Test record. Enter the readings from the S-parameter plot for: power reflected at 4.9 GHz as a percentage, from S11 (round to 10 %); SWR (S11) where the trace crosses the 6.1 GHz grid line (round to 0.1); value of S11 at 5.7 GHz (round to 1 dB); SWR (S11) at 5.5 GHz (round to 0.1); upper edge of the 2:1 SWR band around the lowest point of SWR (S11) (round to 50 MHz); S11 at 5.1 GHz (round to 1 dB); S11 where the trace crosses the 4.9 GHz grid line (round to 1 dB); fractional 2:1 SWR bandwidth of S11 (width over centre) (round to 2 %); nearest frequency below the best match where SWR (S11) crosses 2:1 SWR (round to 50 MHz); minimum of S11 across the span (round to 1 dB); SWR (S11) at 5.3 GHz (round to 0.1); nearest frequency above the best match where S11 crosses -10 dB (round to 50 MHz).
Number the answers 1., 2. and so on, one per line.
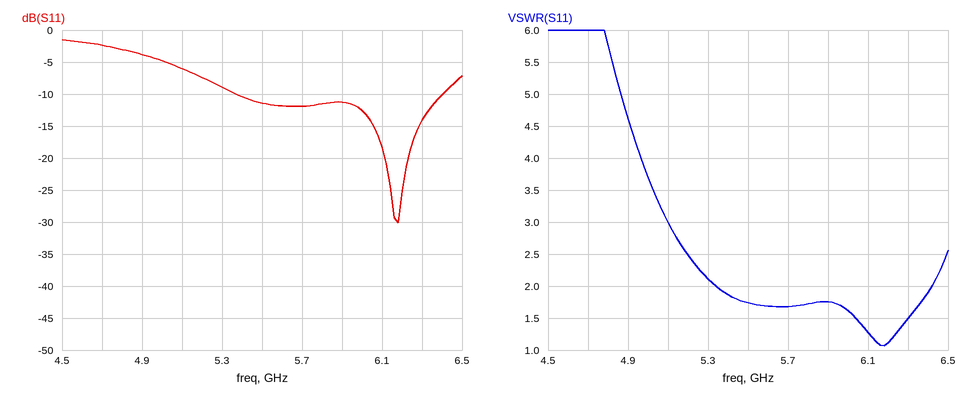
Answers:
1. 40 %
2. 1.3
3. -12 dB
4. 1.7
5. 6.40 GHz
6. -6 dB
7. -4 dB
8. 18 %
9. 5.35 GHz
10. -30 dB
11. 2.1
12. 6.40 GHz
